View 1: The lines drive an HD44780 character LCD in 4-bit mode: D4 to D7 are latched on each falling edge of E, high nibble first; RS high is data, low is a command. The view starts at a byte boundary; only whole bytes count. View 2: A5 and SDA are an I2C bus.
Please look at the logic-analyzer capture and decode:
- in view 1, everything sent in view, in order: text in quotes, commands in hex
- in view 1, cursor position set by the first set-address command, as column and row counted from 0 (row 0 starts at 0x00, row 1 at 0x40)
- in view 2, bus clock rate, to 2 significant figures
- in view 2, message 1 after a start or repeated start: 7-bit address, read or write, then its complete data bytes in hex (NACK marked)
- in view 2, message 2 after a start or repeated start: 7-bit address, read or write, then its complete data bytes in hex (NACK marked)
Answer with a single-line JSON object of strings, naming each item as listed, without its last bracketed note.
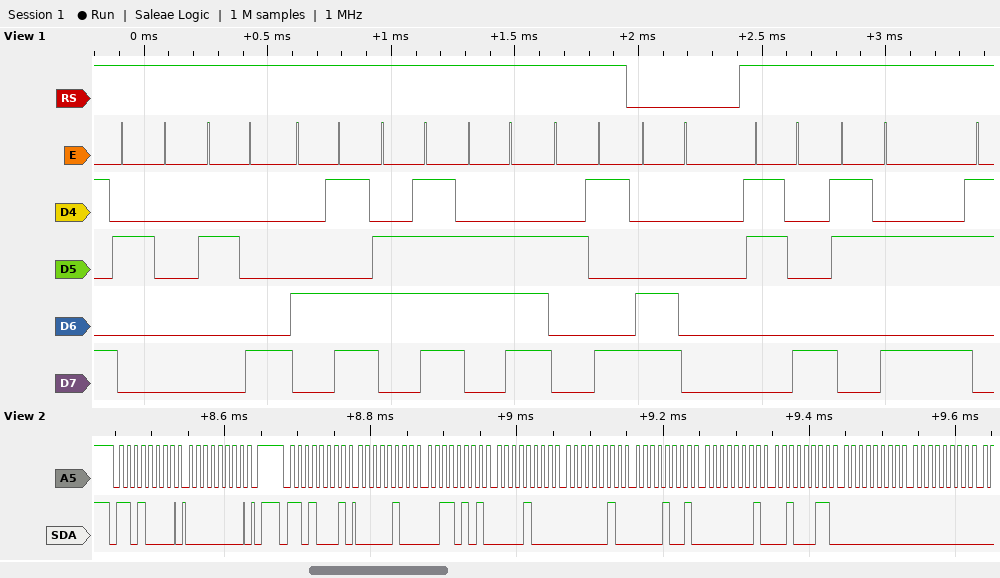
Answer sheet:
{"in view 1, everything sent in view, in order: text in quotes, commands in hex": "\" (Mon)\" 0xC0 \"8:\"", "in view 1, cursor position set by the first set-address command, as column and row counted from 0": "column 0, row 1", "in view 2, bus clock rate, to 2 significant figures": "100 kHz", "in view 2, message 1 after a start or repeated start: 7-bit address, read or write, then its complete data bytes in hex": "0x68 write: 00", "in view 2, message 2 after a start or repeated start: 7-bit address, read or write, then its complete data bytes in hex": "0x68 read: 04 35 08 02 09 01 23 00 00"}
